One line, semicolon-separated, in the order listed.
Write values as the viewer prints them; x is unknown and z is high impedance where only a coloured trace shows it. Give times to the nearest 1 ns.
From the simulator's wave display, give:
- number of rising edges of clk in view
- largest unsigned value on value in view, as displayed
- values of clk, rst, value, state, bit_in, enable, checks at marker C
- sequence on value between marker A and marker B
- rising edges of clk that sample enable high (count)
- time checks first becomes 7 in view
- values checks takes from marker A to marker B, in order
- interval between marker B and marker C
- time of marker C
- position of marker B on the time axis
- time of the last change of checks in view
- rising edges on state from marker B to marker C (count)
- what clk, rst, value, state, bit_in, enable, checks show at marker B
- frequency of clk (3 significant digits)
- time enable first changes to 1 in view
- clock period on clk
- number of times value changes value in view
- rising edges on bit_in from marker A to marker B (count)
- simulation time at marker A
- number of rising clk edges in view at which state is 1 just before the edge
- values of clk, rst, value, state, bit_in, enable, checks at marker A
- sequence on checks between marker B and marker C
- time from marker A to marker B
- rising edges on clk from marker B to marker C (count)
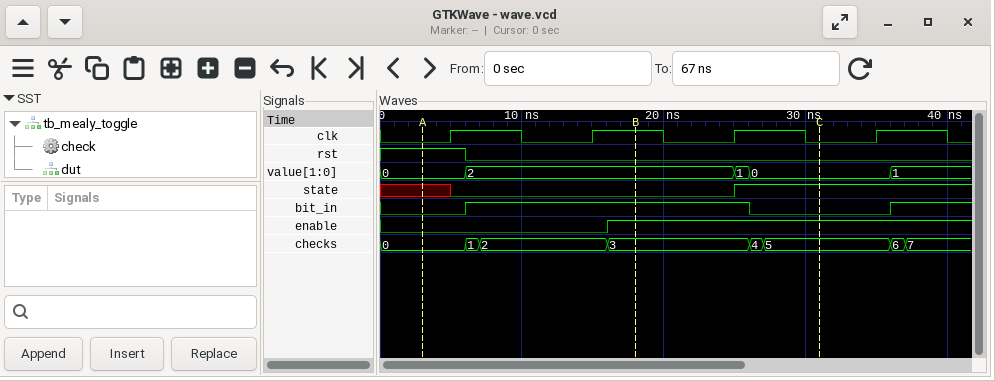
4; 2; clk=0, rst=0, value=0, state=1, bit_in=0, enable=1, checks=5; 0, 2; 2; 37 ns; 0, 1, 2, 3; 13 ns; 31 ns; 18 ns; 37 ns; 1; clk=1, rst=0, value=2, state=0, bit_in=1, enable=1, checks=3; 100 MHz; 16 ns; 10 ns; 4; 1; 3 ns; 1; clk=0, rst=1, value=0, state=x, bit_in=0, enable=0, checks=0; 3, 4, 5; 15 ns; 1
